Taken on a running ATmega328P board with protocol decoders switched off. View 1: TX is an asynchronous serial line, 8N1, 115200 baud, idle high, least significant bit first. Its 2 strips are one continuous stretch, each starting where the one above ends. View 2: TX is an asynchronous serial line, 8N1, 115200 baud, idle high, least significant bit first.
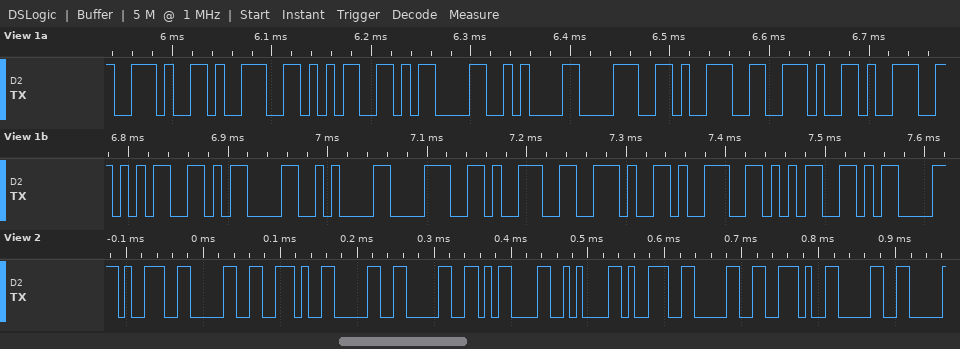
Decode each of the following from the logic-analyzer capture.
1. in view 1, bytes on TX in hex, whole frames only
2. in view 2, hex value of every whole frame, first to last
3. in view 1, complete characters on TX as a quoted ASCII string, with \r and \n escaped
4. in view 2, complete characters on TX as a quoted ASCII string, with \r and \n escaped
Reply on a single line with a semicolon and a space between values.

0x2E 0x39 0x35 0x0D 0x0A 0x38 0x39 0x2E 0x39 0x35 0x0D 0x0A 0x38 0x39 0x2E 0x39 0x35 0x0D; 39 30 2E 30 30 0D 0A 39 30 2E 30; ".95\r\n89.95\r\n89.95\r"; "90.00\r\n90.0"
